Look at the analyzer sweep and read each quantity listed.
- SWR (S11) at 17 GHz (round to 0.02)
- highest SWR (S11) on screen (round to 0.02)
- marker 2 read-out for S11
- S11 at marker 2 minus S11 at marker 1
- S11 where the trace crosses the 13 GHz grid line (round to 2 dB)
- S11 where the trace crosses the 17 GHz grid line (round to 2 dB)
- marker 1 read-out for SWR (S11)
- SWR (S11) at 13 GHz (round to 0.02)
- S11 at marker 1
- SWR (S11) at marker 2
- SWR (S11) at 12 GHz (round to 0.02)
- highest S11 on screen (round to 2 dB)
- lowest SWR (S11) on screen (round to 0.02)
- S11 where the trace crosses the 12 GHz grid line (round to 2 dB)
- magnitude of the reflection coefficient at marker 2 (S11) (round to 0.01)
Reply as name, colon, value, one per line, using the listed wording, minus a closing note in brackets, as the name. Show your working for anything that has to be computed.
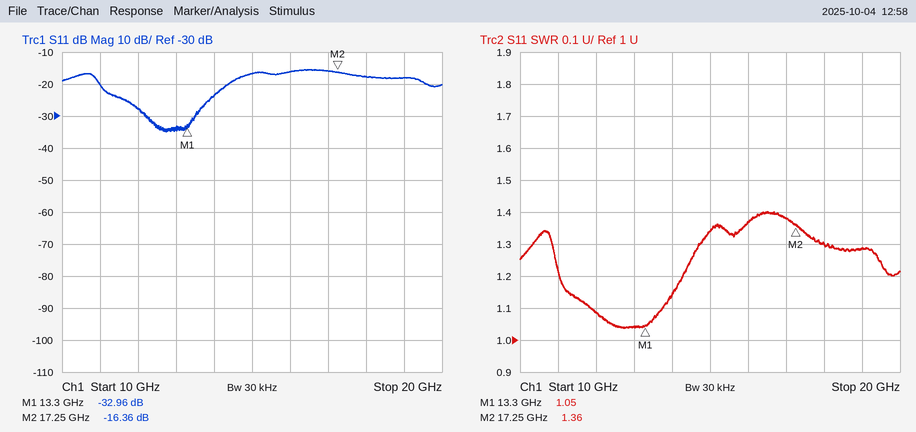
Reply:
SWR (S11) at 17 GHz: 1.38
highest SWR (S11) on screen: 1.40
marker 2 read-out for S11: -16.36 dB
S11 at marker 2 minus S11 at marker 1: -16.36 − (-32.96) = 16.60 dB
S11 where the trace crosses the 13 GHz grid line: -34 dB
S11 where the trace crosses the 17 GHz grid line: -16 dB
marker 1 read-out for SWR: 1.05
SWR (S11) at 13 GHz: 1.04
S11 at marker 1: -32.96 dB
SWR (S11) at marker 2: 1.36
SWR (S11) at 12 GHz: 1.08
highest S11 on screen: -16 dB
lowest SWR (S11) on screen: 1.04
S11 where the trace crosses the 12 GHz grid line: -28 dB
magnitude of the reflection coefficient at marker 2 (S11): 10^(-16.36/20) ≈ 0.15
